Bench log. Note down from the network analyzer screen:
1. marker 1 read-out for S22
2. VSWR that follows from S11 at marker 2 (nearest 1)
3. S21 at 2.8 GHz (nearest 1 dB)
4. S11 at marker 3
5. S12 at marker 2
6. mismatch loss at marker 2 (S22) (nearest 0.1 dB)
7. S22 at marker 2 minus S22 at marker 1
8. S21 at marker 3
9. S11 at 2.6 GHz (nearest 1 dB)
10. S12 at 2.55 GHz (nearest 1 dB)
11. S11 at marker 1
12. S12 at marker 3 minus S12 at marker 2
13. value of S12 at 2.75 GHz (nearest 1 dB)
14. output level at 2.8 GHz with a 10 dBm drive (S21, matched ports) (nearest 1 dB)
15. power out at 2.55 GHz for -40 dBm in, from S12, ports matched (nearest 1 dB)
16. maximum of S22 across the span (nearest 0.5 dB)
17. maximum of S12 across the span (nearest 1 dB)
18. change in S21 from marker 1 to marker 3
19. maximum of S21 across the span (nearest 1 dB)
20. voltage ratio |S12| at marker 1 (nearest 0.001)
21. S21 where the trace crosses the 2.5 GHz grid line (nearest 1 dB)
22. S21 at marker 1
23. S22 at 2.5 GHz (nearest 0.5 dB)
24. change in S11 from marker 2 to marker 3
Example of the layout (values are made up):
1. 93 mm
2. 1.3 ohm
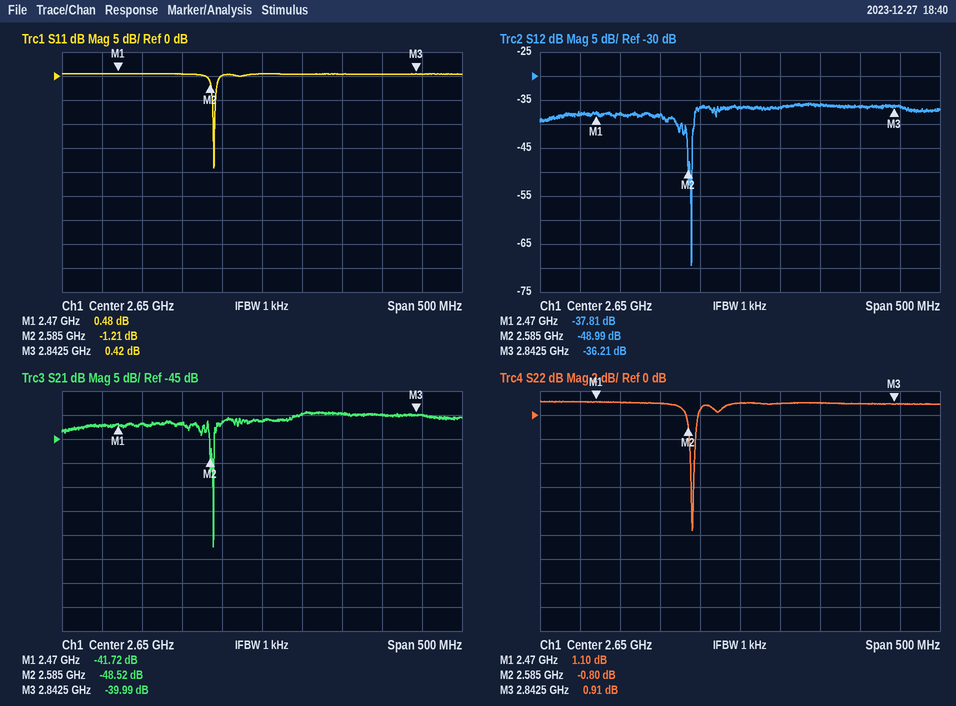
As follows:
1. 1.10 dB
2. 14
3. -40 dB
4. 0.42 dB
5. -48.99 dB
6. 7.7 dB
7. -1.90 dB
8. -39.99 dB
9. 0 dB
10. -38 dB
11. 0.48 dB
12. 12.78 dB
13. -36 dB
14. -30 dBm
15. -78 dBm
16. 1.0 dB
17. -36 dB
18. 1.73 dB
19. -39 dB
20. 0.013
21. -42 dB
22. -41.72 dB
23. 1.0 dB
24. 1.63 dB
